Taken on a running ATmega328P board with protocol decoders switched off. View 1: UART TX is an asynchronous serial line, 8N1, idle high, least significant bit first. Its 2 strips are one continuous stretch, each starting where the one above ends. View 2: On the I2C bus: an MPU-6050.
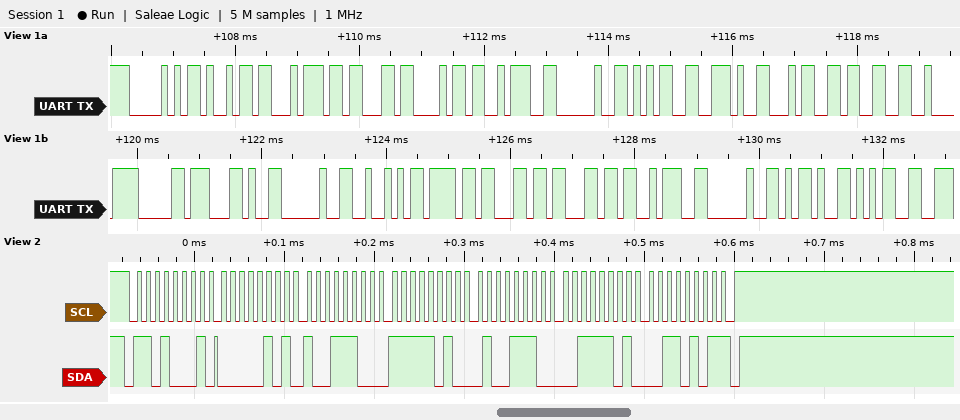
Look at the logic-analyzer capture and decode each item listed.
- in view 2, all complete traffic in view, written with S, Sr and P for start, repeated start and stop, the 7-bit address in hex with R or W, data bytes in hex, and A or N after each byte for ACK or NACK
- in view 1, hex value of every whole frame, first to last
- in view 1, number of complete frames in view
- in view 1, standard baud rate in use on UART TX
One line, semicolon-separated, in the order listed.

S 68R A 05 A 9C A FA A 4E A 3D A 35 N P; 50 69 74 63 68 3A 20 35 2E 34 33 C2 B0 2C 20 52 6F 6C 6C 3A 20 2D 35; 23; 9600 baud
